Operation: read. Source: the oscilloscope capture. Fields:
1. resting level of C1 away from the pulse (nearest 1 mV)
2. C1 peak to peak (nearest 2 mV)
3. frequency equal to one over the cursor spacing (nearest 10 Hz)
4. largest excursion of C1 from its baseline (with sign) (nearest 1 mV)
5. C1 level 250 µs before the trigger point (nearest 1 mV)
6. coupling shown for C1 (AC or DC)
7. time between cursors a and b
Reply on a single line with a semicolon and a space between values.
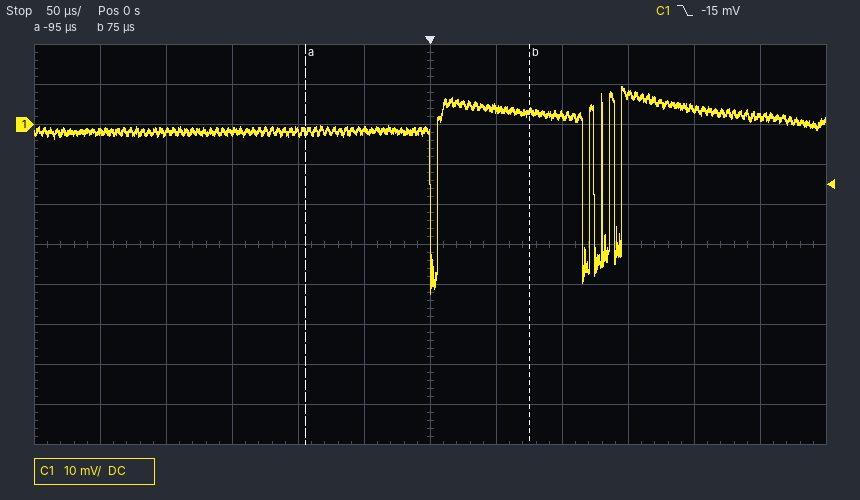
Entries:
-2 mV; 52 mV; 5.88 kHz; -41 mV; -2 mV; DC; 170 µs
